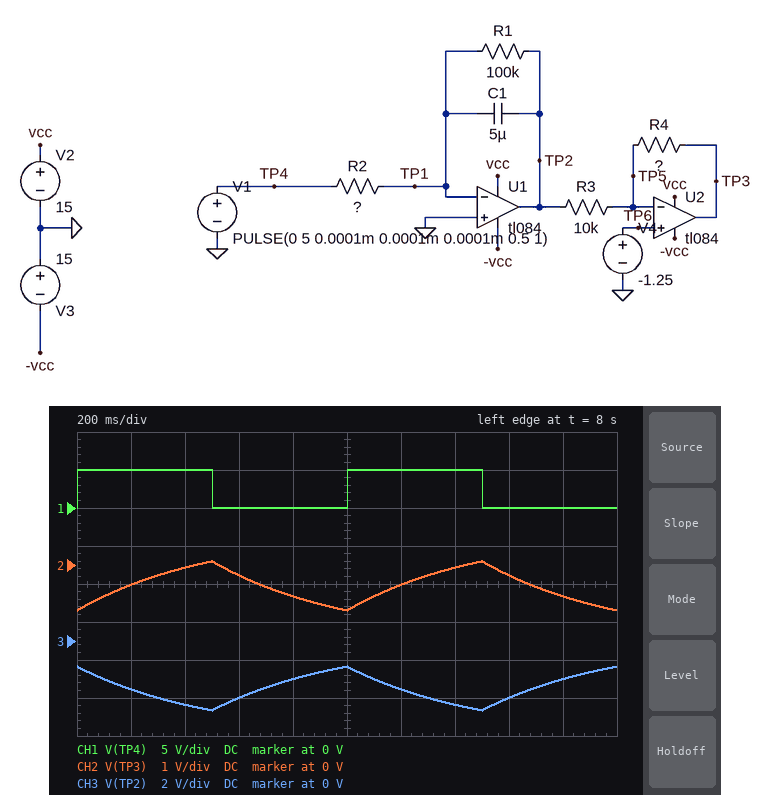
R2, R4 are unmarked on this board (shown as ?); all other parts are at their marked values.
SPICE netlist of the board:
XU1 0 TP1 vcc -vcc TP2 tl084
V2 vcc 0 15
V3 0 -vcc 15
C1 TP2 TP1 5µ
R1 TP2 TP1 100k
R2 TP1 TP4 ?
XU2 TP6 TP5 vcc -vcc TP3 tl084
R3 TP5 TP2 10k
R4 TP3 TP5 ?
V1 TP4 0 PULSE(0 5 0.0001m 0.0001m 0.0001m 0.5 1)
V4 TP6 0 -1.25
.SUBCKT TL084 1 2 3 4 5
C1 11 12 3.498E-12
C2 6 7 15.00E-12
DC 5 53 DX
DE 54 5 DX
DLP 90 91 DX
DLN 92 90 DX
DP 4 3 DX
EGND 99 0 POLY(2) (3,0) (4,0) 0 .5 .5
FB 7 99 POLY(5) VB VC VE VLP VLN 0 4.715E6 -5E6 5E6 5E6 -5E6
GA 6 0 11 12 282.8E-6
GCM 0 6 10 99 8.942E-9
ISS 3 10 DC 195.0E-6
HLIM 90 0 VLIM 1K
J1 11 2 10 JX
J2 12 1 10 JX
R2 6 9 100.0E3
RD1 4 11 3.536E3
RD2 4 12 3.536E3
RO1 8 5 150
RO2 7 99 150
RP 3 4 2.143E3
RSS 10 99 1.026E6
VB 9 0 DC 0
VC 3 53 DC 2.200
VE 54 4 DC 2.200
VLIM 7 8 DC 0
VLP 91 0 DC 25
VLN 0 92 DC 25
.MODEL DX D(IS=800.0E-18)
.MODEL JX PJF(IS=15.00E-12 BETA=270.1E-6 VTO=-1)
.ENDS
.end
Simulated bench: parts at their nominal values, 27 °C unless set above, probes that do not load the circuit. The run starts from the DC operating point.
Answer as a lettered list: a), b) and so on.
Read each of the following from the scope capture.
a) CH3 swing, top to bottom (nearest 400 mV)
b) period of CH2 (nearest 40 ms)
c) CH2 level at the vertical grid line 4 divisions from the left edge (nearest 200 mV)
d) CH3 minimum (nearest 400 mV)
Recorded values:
a) 2.4 V
b) 1.00 s
c) -800 mV
d) -3.6 V
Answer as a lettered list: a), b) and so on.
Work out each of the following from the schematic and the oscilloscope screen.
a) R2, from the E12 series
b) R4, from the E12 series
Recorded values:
a) 100 kΩ
b) 5.6 kΩ
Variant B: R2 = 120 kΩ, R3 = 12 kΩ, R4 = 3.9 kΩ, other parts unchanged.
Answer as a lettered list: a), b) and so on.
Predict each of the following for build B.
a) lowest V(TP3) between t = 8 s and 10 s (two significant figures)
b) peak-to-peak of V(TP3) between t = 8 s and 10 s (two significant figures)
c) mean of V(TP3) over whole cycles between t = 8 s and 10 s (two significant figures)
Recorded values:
a) -1.3 V
b) 630 mV
c) -980 mV
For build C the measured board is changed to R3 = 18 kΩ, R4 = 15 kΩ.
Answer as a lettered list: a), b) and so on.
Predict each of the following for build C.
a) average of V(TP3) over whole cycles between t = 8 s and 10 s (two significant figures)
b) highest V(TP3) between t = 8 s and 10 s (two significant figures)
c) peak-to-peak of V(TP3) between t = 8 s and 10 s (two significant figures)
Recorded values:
a) -210 mV
b) 760 mV
c) 1.9 V
